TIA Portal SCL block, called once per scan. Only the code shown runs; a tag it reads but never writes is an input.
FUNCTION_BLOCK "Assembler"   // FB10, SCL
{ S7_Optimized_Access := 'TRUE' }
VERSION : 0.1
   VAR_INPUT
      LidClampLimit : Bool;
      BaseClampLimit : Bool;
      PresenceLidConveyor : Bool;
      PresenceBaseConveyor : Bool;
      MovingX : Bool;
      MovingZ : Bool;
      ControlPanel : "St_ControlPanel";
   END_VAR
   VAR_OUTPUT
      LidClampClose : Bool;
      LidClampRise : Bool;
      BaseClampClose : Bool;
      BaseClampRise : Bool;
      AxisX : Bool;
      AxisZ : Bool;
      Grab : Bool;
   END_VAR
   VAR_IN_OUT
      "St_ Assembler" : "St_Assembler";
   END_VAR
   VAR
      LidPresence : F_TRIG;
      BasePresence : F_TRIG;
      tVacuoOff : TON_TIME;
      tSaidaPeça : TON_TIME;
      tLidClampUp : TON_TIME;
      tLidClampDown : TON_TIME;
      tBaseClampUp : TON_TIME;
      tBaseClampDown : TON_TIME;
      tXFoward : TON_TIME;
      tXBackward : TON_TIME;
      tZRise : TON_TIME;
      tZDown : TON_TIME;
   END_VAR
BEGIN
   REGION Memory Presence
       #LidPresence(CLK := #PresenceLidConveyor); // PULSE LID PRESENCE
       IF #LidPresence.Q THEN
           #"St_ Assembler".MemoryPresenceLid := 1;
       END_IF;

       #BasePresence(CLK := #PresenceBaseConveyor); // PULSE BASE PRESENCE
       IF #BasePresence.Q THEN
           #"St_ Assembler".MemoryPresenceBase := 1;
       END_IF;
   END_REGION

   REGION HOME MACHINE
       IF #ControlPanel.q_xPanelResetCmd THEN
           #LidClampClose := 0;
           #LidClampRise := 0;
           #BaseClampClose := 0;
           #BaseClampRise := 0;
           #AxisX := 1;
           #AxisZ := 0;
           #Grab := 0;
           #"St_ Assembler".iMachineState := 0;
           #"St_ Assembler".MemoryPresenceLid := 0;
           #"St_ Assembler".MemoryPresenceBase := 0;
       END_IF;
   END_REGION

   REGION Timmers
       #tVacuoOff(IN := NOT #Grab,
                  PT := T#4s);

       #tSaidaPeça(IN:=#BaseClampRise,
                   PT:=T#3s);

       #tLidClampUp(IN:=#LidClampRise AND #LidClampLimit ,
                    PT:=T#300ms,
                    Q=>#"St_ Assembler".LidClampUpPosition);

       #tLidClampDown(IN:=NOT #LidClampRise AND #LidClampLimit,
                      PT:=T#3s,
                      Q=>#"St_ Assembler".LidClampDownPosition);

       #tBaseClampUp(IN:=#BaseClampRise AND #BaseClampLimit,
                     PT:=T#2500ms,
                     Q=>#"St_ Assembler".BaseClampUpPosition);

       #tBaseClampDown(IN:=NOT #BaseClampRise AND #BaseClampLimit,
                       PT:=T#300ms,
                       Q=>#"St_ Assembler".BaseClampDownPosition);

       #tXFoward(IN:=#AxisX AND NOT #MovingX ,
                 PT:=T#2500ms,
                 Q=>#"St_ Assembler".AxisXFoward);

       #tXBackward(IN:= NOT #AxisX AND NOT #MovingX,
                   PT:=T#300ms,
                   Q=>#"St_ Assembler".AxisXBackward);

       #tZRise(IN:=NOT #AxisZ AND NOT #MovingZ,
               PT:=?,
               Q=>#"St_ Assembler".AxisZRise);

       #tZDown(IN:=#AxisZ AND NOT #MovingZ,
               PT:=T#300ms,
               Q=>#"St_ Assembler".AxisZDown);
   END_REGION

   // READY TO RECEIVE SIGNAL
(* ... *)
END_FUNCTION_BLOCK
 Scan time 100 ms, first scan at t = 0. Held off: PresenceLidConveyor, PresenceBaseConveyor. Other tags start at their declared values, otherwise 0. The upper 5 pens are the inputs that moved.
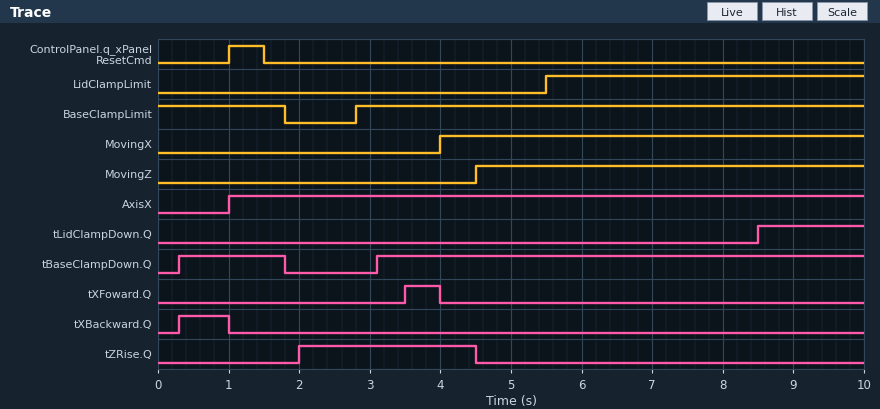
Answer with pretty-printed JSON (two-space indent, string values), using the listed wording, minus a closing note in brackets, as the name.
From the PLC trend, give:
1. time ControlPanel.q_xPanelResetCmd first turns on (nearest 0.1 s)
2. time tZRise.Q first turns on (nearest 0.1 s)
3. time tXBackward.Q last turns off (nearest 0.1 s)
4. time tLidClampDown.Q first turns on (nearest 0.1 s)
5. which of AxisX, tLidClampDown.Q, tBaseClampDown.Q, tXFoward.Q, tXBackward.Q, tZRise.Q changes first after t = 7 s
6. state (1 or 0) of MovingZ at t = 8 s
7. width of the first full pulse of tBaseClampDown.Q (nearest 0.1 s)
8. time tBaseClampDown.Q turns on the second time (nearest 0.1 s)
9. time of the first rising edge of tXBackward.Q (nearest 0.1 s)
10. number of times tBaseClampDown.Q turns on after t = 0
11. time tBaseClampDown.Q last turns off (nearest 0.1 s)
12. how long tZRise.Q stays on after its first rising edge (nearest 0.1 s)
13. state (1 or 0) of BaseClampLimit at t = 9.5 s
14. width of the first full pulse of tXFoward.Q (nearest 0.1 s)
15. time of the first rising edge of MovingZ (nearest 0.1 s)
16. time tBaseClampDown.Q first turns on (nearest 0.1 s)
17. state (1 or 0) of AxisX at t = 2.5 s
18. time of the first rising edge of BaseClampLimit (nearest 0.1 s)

{
  "time ControlPanel.q_xPanelResetCmd first turns on": "1.0 s",
  "time tZRise.Q first turns on": "2.0 s",
  "time tXBackward.Q last turns off": "1.0 s",
  "time tLidClampDown.Q first turns on": "8.5 s",
  "which of AxisX, tLidClampDown.Q, tBaseClampDown.Q, tXFoward.Q, tXBackward.Q, tZRise.Q changes first after t = 7 s": "tLidClampDown.Q",
  "state (1 or 0) of MovingZ at t = 8 s": "1",
  "width of the first full pulse of tBaseClampDown.Q": "1.5 s",
  "time tBaseClampDown.Q turns on the second time": "3.1 s",
  "time of the first rising edge of tXBackward.Q": "0.3 s",
  "number of times tBaseClampDown.Q turns on after t = 0": "2",
  "time tBaseClampDown.Q last turns off": "1.8 s",
  "how long tZRise.Q stays on after its first rising edge": "2.5 s",
  "state (1 or 0) of BaseClampLimit at t = 9.5 s": "1",
  "width of the first full pulse of tXFoward.Q": "0.5 s",
  "time of the first rising edge of MovingZ": "4.5 s",
  "time tBaseClampDown.Q first turns on": "0.3 s",
  "state (1 or 0) of AxisX at t = 2.5 s": "1",
  "time of the first rising edge of BaseClampLimit": "2.8 s"
}
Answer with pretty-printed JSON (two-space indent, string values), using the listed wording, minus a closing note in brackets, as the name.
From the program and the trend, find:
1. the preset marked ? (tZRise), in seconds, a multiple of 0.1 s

{
  "the preset marked ? (tZRise), in seconds, a multiple of 0.1 s": "2.0 s"
}
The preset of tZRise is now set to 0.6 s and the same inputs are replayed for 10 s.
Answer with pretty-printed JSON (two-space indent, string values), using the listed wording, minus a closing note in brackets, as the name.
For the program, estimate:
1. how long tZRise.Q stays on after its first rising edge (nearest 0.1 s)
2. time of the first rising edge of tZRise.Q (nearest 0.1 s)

{
  "how long tZRise.Q stays on after its first rising edge": "3.9 s",
  "time of the first rising edge of tZRise.Q": "0.6 s"
}
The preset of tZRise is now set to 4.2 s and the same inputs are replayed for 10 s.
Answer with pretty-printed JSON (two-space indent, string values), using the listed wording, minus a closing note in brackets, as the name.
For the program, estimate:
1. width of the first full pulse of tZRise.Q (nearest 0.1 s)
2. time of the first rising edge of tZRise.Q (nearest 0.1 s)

{
  "width of the first full pulse of tZRise.Q": "0.3 s",
  "time of the first rising edge of tZRise.Q": "4.2 s"
}
